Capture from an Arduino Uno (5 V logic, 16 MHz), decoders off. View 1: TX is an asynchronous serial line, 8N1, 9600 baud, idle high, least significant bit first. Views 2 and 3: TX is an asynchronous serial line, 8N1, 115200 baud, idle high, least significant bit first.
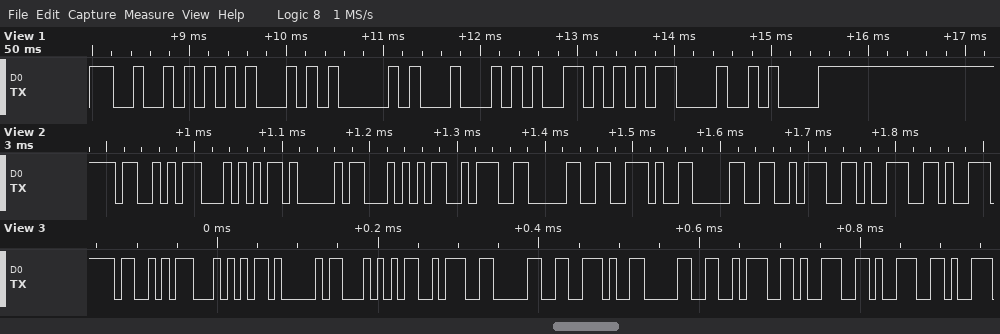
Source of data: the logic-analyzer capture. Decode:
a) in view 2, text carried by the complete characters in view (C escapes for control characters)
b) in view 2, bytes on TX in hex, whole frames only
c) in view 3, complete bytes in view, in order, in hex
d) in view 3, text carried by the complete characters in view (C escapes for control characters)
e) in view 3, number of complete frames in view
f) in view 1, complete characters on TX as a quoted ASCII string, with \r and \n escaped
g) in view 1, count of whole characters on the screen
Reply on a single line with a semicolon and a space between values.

"STAT:0.0:9"; 53 54 41 54 3A 30 2E 30 3A 39; 53 54 41 54 3A 30 2E 30 3A 39 39; "STAT:0.0:99"; 11; "READY\r\n"; 7
